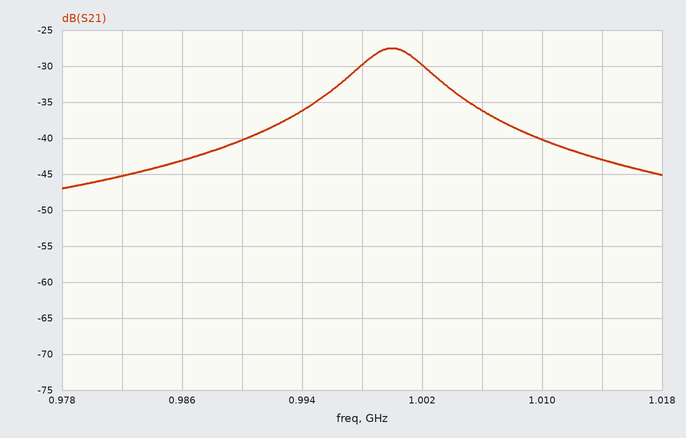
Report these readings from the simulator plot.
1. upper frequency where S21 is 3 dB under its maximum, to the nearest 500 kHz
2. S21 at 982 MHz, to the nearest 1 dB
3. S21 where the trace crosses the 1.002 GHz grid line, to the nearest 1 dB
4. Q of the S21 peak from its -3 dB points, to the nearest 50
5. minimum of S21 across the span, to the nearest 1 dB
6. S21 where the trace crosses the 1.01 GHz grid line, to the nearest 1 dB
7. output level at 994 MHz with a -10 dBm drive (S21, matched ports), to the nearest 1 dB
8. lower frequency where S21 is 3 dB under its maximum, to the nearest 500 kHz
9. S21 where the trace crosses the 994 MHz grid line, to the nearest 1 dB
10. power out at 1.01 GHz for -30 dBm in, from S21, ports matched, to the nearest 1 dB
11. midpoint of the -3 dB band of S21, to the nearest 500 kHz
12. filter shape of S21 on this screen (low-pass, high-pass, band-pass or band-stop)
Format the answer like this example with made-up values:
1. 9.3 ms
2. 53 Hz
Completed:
1. 1.0025 GHz
2. -45 dB
3. -30 dB
4. 200
5. -47 dB
6. -40 dB
7. -46 dBm
8. 997.5 MHz
9. -36 dB
10. -70 dBm
11. 1.0000 GHz
12. band-pass
